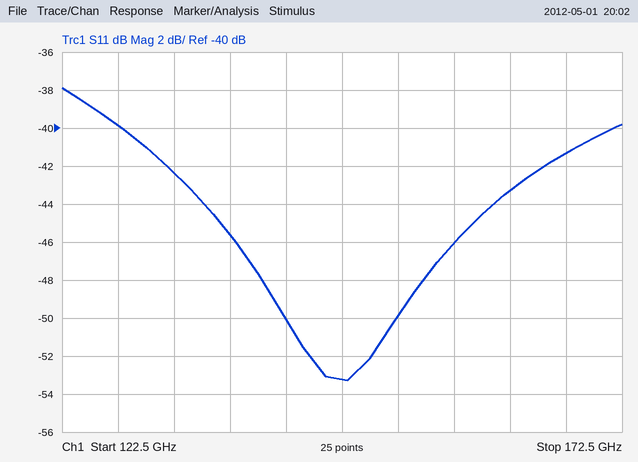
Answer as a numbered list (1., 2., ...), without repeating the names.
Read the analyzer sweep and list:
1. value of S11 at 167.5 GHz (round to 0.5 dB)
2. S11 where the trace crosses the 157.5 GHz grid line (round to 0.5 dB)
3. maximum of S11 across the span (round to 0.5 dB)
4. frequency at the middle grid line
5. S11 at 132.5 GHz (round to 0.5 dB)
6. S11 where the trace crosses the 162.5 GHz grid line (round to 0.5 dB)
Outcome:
1. -41.5 dB
2. -46.0 dB
3. -38.0 dB
4. 147.5 GHz
5. -42.5 dB
6. -43.5 dB
